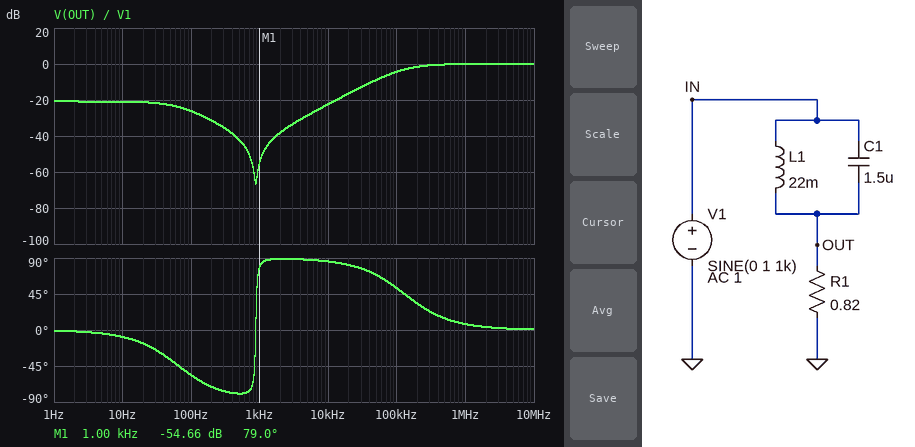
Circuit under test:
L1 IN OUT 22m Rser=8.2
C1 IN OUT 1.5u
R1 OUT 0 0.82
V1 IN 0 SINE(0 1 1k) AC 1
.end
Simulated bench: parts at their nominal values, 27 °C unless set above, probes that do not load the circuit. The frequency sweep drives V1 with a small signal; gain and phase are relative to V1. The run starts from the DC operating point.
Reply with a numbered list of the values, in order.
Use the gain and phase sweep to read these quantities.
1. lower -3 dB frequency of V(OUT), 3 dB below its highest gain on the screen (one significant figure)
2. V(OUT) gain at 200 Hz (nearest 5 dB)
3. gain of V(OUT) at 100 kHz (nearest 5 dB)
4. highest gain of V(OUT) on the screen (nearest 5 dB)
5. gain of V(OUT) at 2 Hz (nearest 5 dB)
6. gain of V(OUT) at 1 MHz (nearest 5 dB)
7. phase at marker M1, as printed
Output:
1. 100 kHz
2. -30 dB
3. -5 dB
4. 0 dB
5. -20 dB
6. 0 dB
7. 79.0 deg
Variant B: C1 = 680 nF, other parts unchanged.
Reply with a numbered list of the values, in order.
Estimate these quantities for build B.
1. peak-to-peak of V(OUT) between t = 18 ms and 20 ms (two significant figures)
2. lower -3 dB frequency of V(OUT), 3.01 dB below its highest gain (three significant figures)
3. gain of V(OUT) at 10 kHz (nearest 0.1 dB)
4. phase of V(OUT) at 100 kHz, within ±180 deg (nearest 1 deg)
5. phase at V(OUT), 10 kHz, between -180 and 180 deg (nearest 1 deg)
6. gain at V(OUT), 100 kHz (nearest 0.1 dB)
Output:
1. 4.9 mV
2. 285 kHz
3. -29.3 dB
4. 71 deg
5. 88 deg
6. -9.6 dB
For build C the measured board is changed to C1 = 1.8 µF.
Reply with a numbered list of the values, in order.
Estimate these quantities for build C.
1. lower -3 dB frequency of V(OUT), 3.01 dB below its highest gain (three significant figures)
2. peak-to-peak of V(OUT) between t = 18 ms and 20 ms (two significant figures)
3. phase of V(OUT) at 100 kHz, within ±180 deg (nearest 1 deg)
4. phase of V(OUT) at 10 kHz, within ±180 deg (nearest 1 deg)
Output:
1. 108 kHz
2. 6.8 mV
3. 47 deg
4. 85 deg
